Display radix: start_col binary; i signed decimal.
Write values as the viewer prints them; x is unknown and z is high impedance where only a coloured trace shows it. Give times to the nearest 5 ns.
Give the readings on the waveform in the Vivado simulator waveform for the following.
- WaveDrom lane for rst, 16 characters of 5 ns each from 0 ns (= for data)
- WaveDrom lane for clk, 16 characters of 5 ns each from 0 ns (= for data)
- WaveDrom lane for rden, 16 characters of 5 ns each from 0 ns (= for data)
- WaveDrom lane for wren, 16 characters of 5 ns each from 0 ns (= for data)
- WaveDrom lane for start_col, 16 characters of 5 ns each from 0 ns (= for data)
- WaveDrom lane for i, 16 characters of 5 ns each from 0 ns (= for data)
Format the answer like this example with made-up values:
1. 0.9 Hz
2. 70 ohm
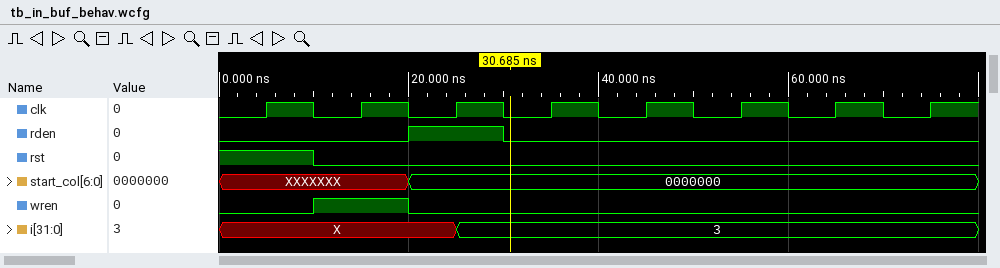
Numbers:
1. {name: 'rst', wave: '1.0.............'}
2. {name: 'clk', wave: '0101010101010101'}
3. {name: 'rden', wave: '0...1.0.........'}
4. {name: 'wren', wave: '0.1.0...........'}
5. {name: 'start_col', wave: 'x...=...........', data: '0000000'}
6. {name: 'i', wave: 'x....=..........', data: '3'}
